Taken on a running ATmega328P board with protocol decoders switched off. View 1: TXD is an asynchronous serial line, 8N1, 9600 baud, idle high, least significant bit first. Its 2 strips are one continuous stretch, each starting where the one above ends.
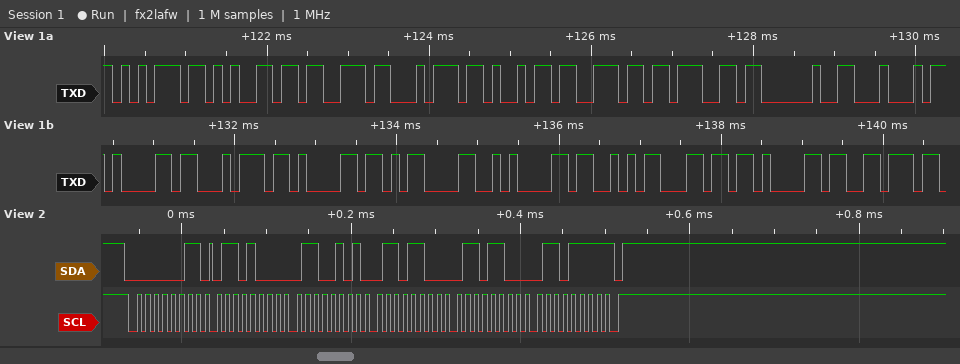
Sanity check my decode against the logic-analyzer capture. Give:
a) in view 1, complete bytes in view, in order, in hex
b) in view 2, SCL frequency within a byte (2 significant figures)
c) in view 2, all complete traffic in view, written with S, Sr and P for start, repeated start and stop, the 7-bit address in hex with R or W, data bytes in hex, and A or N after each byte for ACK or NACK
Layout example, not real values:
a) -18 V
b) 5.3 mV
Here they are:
a) 75 65 73 74 69 6E 67 20 44 61 74 61 0D 0A 53 6C 61 76
b) 100 kHz
c) S 01R A 68 A 65 A 6C A 6C A 6F N P
